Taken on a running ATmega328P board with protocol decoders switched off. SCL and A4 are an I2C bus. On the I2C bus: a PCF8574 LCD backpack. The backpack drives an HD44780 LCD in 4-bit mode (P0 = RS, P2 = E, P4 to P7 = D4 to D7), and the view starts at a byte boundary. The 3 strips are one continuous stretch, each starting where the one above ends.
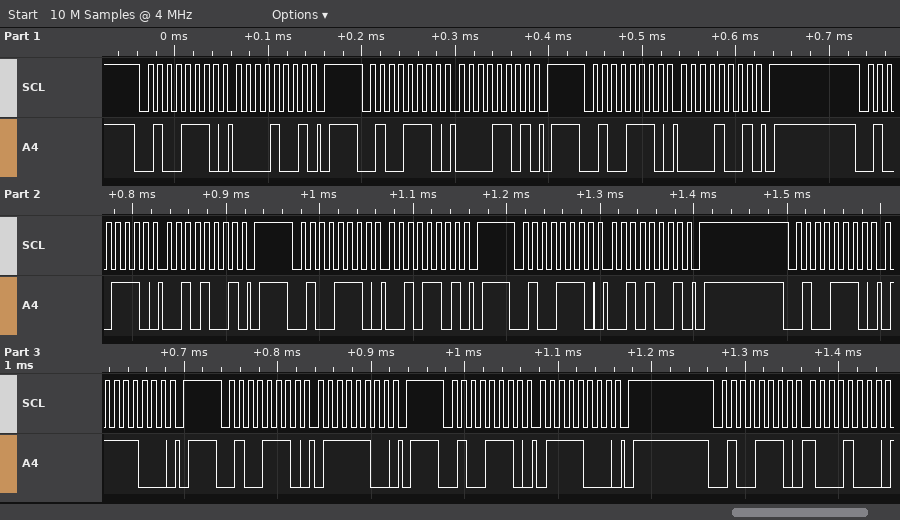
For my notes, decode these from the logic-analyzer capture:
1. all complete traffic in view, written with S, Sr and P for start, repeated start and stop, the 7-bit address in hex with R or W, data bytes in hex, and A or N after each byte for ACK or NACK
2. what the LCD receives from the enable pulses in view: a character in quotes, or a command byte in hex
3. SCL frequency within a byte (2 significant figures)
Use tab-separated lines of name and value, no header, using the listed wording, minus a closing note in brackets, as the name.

all complete traffic in view, written with S, Sr and P for start, repeated start and stop, the 7-bit address in hex with R or W, data bytes in hex, and A or N after each byte for ACK or NACK	S 27W A 09 A P S 27W A 0D A P S 27W A 09 A P S 27W A 29 A P S 27W A 2D A P S 27W A 29 A P S 27W A 78 A P S 27W A 7C A P S 27W A 78 A P S 27W A 88 A
what the LCD receives from the enable pulses in view: a character in quotes, or a command byte in hex	data 0x02
SCL frequency within a byte	100 kHz
